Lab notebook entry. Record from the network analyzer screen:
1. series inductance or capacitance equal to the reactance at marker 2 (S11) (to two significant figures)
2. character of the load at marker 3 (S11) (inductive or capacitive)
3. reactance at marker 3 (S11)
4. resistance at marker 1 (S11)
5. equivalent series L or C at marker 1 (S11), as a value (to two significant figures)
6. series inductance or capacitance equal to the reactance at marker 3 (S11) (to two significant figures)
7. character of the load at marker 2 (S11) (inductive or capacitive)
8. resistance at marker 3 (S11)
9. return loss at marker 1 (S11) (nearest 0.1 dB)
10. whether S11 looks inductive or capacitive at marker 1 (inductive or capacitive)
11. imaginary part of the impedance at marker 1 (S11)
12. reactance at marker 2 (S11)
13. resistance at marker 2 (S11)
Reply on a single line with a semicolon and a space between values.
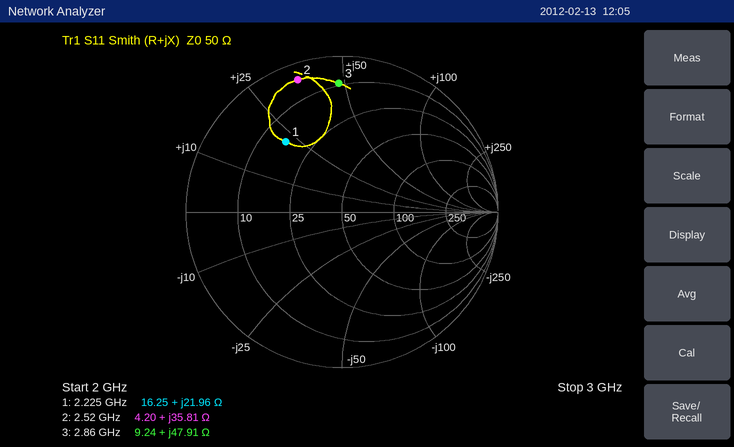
2.3 nH; inductive; +47.91 Ω; 16.25 Ω; 1.6 nH; 2.7 nH; inductive; 9.24 Ω; 4.8 dB; inductive; +21.96 Ω; +35.81 Ω; 4.20 Ω
